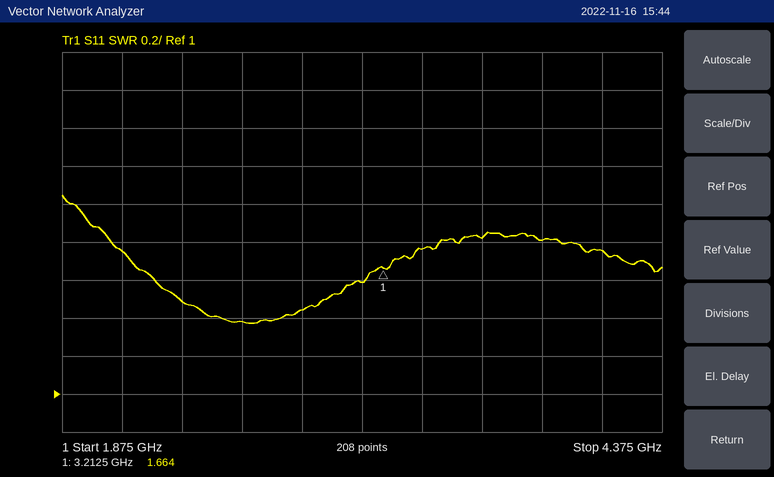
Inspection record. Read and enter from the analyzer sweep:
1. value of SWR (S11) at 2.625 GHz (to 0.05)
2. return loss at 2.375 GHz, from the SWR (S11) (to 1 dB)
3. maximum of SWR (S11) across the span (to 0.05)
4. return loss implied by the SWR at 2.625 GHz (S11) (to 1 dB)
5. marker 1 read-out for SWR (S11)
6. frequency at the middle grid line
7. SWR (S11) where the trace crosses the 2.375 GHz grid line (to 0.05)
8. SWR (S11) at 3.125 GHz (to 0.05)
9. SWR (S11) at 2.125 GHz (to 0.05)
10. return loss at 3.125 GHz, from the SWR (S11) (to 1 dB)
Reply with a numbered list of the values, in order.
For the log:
1. 1.40
2. 14 dB
3. 2.05
4. 16 dB
5. 1.664
6. 3.125 GHz
7. 1.50
8. 1.60
9. 1.75
10. 13 dB
